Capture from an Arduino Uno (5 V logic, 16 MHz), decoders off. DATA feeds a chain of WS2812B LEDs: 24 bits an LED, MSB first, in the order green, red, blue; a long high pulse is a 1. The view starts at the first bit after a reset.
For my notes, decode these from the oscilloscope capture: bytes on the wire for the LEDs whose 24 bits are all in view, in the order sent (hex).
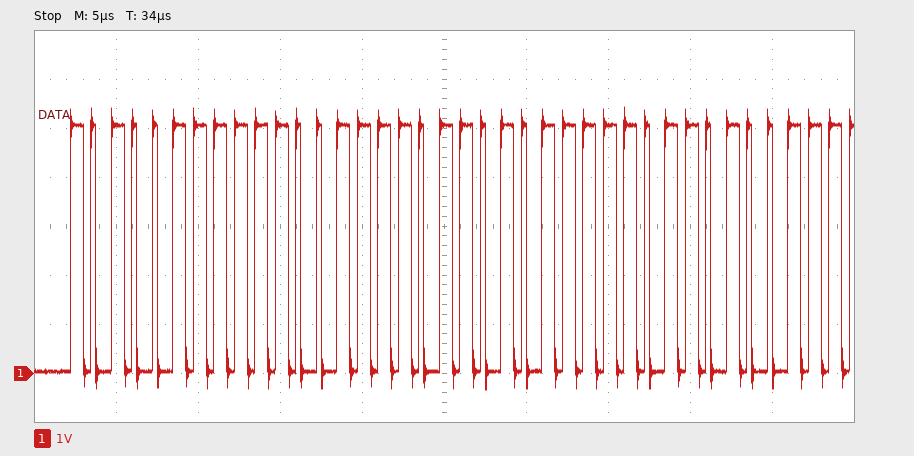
A7 E7 B5
